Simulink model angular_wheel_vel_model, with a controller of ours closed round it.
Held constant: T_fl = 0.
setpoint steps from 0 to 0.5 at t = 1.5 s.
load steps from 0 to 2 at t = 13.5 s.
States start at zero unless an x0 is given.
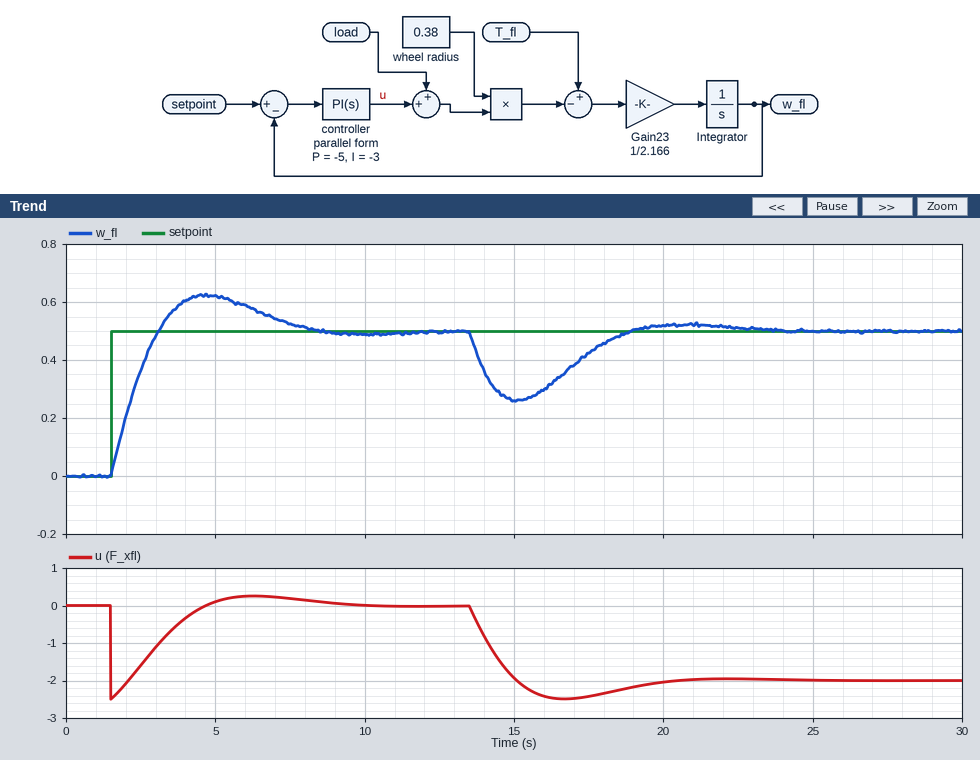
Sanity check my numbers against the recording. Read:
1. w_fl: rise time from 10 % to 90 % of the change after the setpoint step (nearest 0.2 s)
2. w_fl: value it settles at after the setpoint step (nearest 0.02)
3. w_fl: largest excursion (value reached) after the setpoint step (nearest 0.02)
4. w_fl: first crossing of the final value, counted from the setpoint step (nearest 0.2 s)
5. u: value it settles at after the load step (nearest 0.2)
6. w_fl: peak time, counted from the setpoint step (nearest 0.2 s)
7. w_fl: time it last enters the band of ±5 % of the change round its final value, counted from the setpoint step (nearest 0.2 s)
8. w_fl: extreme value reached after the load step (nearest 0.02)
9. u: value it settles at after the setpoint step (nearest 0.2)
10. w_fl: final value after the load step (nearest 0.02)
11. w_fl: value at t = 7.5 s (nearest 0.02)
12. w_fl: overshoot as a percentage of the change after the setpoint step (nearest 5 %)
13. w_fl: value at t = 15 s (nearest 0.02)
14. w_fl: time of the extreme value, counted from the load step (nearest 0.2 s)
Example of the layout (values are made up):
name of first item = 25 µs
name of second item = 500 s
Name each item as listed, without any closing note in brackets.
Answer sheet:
w_fl: rise time from 10 % to 90 % of the change after the setpoint step = 1.2 s
w_fl: value it settles at after the setpoint step = 0.50
w_fl: largest excursion (value reached) after the setpoint step = 0.62
w_fl: first crossing of the final value, counted from the setpoint step = 1.6 s
u: value it settles at after the load step = -2.0
w_fl: peak time, counted from the setpoint step = 3.2 s
w_fl: time it last enters the band of ±5 % of the change round its final value, counted from the setpoint step = 6.0 s
w_fl: extreme value reached after the load step = 0.26
u: value it settles at after the setpoint step = 0.0
w_fl: final value after the load step = 0.50
w_fl: value at t = 7.5 s = 0.52
w_fl: overshoot as a percentage of the change after the setpoint step = 25 %
w_fl: value at t = 15 s = 0.26
w_fl: time of the extreme value, counted from the load step = 1.6 s
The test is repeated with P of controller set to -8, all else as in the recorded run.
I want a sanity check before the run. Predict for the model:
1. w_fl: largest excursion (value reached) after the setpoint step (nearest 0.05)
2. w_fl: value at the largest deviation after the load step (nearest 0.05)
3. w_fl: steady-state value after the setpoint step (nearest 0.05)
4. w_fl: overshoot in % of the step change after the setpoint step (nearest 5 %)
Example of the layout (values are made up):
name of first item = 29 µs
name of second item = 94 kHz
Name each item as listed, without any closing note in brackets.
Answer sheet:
w_fl: largest excursion (value reached) after the setpoint step = 0.55
w_fl: value at the largest deviation after the load step = 0.30
w_fl: steady-state value after the setpoint step = 0.50
w_fl: overshoot in % of the step change after the setpoint step = 15 %
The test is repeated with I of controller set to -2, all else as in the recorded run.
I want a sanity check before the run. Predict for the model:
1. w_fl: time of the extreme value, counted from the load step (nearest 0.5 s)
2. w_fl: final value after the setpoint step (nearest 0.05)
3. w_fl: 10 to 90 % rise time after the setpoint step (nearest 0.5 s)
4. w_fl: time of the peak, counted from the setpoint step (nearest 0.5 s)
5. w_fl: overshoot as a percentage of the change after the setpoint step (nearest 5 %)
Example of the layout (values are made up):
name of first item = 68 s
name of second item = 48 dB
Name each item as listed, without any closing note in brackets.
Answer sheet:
w_fl: time of the extreme value, counted from the load step = 2.0 s
w_fl: final value after the setpoint step = 0.50
w_fl: 10 to 90 % rise time after the setpoint step = 1.5 s
w_fl: time of the peak, counted from the setpoint step = 3.5 s
w_fl: overshoot as a percentage of the change after the setpoint step = 20 %
